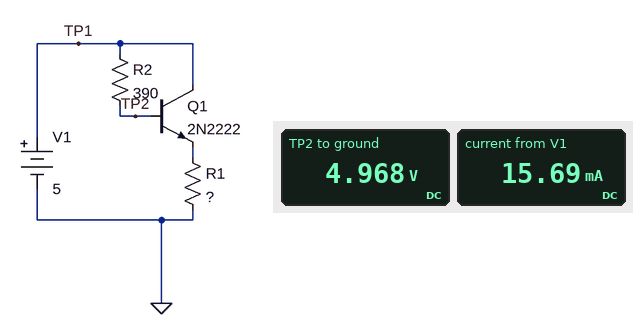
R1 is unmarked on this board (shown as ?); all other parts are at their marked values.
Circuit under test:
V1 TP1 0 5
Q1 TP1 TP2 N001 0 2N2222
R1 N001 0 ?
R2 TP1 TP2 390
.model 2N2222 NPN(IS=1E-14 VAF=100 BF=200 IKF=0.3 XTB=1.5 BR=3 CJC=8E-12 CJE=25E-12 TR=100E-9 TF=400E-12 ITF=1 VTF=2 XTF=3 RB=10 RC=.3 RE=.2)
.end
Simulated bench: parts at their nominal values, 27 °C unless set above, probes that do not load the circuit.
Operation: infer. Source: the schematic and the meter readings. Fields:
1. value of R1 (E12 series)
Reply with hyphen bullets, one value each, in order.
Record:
- 270 Ω
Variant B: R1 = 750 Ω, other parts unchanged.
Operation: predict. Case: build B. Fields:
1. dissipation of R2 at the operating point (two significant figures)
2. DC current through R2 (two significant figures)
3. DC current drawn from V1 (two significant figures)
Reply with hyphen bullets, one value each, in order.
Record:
- 330 nW
- 29 µA
- 5.7 mA
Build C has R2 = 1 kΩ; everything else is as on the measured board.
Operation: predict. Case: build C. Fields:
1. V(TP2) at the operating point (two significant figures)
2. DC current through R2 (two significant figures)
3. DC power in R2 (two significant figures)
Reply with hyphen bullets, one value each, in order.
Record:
- 4.9 V
- 81 µA
- 6.6 µW
